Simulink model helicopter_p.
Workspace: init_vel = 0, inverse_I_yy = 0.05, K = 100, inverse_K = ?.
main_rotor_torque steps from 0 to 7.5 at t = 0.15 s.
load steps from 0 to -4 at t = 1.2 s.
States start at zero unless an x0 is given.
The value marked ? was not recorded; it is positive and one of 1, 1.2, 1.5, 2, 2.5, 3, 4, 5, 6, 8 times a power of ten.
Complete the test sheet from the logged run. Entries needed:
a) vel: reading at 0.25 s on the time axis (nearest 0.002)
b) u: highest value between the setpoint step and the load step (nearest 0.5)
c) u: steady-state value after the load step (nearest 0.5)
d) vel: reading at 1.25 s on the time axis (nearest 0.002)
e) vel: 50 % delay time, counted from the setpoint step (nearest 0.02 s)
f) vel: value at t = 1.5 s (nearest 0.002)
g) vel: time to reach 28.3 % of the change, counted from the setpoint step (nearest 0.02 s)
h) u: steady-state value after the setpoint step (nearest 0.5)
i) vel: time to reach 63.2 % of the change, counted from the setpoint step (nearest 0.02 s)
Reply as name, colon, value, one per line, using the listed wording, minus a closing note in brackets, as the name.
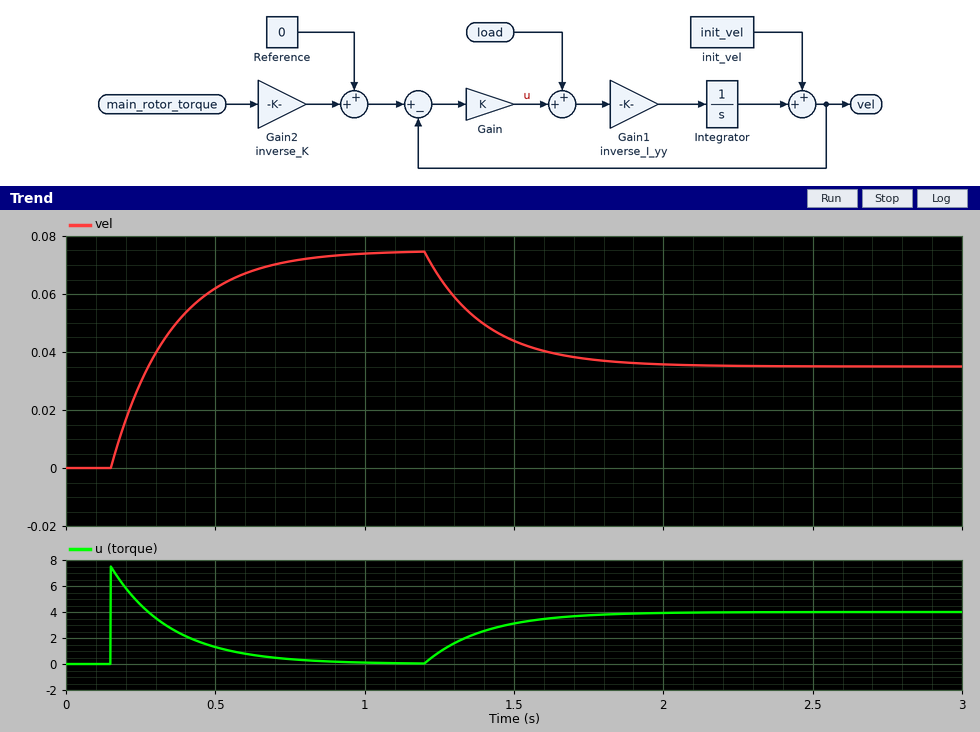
vel: reading at 0.25 s on the time axis: 0.030
u: highest value between the setpoint step and the load step: 7.5
u: steady-state value after the load step: 4.0
vel: reading at 1.25 s on the time axis: 0.066
vel: 50 % delay time, counted from the setpoint step: 0.14 s
vel: value at t = 1.5 s: 0.044
vel: time to reach 28.3 % of the change, counted from the setpoint step: 0.06 s
u: steady-state value after the setpoint step: 0.0
vel: time to reach 63.2 % of the change, counted from the setpoint step: 0.20 s
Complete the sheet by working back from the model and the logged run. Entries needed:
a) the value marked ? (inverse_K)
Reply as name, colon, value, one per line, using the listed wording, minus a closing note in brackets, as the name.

the value marked ?: 0.01
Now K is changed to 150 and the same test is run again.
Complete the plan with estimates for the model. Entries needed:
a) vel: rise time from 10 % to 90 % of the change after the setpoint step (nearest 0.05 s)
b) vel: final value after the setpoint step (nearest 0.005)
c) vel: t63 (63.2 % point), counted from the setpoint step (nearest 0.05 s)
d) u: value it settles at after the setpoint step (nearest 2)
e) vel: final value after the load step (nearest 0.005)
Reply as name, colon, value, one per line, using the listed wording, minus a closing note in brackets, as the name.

vel: rise time from 10 % to 90 % of the change after the setpoint step: 0.30 s
vel: final value after the setpoint step: 0.075
vel: t63 (63.2 % point), counted from the setpoint step: 0.15 s
u: value it settles at after the setpoint step: 0
vel: final value after the load step: 0.050
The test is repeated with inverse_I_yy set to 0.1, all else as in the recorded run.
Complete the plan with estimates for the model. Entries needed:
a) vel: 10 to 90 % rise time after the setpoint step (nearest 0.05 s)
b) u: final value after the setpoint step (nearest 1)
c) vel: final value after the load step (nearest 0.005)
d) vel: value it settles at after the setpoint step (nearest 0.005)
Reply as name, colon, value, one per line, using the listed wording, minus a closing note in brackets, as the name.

vel: 10 to 90 % rise time after the setpoint step: 0.20 s
u: final value after the setpoint step: 0
vel: final value after the load step: 0.035
vel: value it settles at after the setpoint step: 0.075
